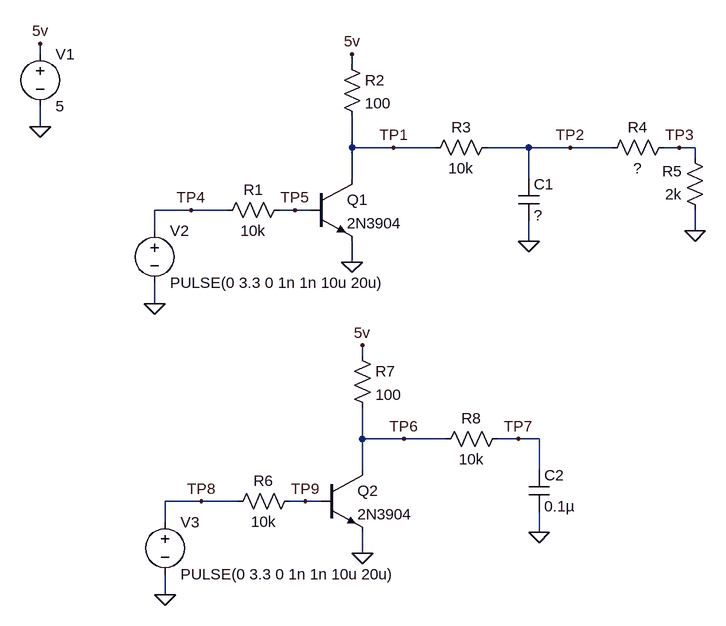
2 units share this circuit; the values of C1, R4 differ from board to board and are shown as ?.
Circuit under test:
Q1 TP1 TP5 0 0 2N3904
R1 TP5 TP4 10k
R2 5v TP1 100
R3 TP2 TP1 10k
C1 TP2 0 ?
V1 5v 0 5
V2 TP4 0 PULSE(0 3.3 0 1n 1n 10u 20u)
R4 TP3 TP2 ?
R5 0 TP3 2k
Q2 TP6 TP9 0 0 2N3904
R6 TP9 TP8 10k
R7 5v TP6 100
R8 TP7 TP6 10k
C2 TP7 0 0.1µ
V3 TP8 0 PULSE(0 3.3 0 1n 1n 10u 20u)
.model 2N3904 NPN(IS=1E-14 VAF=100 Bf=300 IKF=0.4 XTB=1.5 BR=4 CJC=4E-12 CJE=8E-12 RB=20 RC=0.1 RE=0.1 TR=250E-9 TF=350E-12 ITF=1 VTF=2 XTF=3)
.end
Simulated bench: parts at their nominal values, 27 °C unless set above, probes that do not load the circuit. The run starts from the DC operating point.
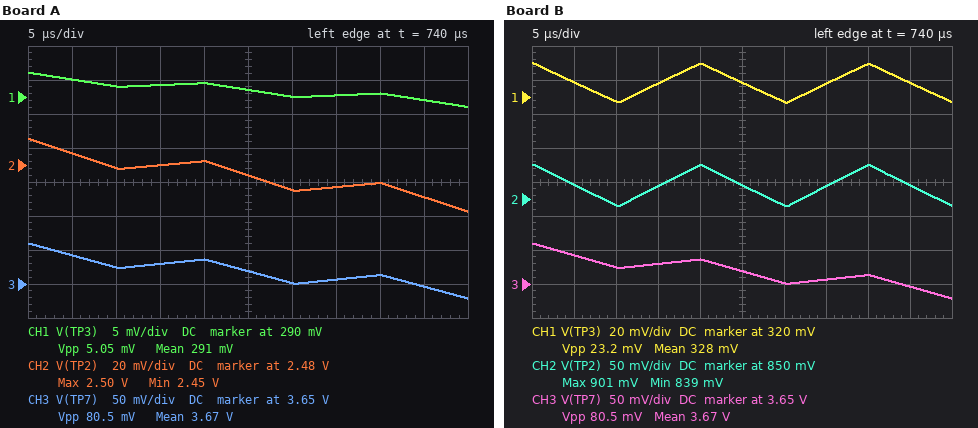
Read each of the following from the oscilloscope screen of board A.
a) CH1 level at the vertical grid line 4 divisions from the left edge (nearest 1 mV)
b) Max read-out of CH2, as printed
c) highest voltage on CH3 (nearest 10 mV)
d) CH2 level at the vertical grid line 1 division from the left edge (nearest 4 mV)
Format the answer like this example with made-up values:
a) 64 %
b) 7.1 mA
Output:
a) 292 mV
b) 2.50 V
c) 3.71 V
d) 2.488 V
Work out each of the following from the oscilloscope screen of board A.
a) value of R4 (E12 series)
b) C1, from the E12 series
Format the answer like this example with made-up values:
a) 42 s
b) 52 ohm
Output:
a) 15 kΩ
b) 220 nF
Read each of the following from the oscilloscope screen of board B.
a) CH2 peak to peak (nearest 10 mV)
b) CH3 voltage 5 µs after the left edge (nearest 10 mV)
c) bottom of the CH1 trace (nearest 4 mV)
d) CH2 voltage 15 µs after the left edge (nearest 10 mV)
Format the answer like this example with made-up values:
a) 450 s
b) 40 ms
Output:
a) 60 mV
b) 3.69 V
c) 316 mV
d) 870 mV
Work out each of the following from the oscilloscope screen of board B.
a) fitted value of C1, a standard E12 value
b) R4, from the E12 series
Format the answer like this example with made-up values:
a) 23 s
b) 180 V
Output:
a) 39 nF
b) 3.3 kΩ
